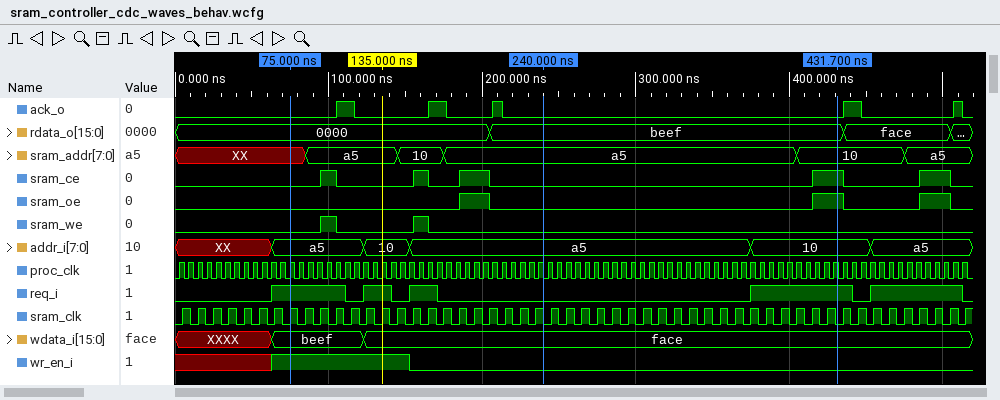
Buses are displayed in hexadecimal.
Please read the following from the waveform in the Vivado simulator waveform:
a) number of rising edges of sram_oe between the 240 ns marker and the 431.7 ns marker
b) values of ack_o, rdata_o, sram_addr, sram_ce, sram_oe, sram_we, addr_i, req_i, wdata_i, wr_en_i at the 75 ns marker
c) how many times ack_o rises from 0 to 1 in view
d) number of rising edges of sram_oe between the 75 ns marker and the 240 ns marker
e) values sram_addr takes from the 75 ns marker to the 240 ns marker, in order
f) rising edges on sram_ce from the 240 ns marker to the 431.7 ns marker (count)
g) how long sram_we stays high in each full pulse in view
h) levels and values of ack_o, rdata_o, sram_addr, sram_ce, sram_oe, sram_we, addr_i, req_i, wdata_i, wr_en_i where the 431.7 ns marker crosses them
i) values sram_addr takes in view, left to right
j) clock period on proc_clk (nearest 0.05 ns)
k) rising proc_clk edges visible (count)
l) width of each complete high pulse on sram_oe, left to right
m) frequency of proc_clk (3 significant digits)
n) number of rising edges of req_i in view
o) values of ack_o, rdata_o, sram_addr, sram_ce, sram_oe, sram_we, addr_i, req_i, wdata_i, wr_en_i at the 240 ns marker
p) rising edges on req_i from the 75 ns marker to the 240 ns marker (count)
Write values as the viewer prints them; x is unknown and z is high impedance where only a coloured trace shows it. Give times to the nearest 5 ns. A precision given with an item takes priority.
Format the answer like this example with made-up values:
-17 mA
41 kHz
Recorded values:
1
ack_o=0, rdata_o=0000, sram_addr=XX, sram_ce=0, sram_oe=0, sram_we=0, addr_i=a5, req_i=1, wdata_i=beef, wr_en_i=1
5
1
XX, a5, 10, a5
1
10 ns, 10 ns
ack_o=0, rdata_o=beef, sram_addr=10, sram_ce=1, sram_oe=1, sram_we=0, addr_i=10, req_i=1, wdata_i=face, wr_en_i=0
XX, a5, 10, a5, 10, a5
6 ns
86
20 ns, 20 ns, 20 ns
167 MHz
5
ack_o=0, rdata_o=beef, sram_addr=a5, sram_ce=0, sram_oe=0, sram_we=0, addr_i=a5, req_i=0, wdata_i=face, wr_en_i=0
2
